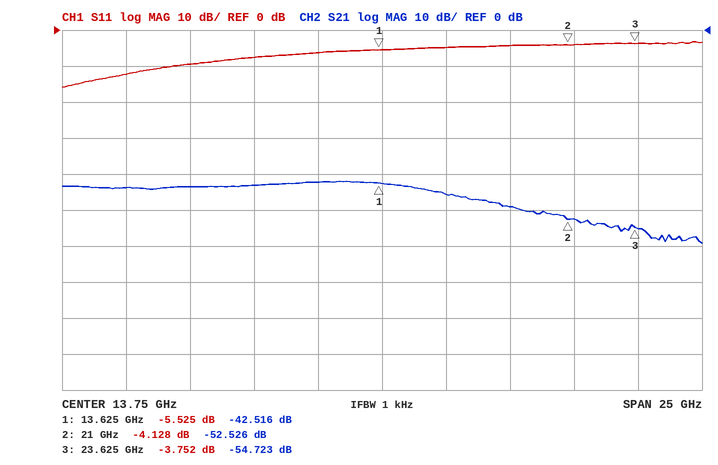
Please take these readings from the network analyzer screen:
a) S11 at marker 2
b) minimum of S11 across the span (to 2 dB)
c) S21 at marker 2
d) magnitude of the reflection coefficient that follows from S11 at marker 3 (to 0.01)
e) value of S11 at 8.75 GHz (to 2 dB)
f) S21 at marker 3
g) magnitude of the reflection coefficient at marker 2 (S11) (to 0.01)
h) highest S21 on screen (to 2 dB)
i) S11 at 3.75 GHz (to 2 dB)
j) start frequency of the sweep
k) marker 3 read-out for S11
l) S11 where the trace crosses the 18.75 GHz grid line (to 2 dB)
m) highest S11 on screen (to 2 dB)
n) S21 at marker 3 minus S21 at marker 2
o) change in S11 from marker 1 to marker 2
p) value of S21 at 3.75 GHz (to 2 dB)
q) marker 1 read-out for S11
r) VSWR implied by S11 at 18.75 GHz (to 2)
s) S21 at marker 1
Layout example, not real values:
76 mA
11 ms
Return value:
-4.128 dB
-16 dB
-52.526 dB
0.65
-8 dB
-54.723 dB
0.62
-42 dB
-12 dB
1.25 GHz
-3.752 dB
-4 dB
-4 dB
-2.197 dB
1.397 dB
-44 dB
-5.525 dB
4
-42.516 dB
